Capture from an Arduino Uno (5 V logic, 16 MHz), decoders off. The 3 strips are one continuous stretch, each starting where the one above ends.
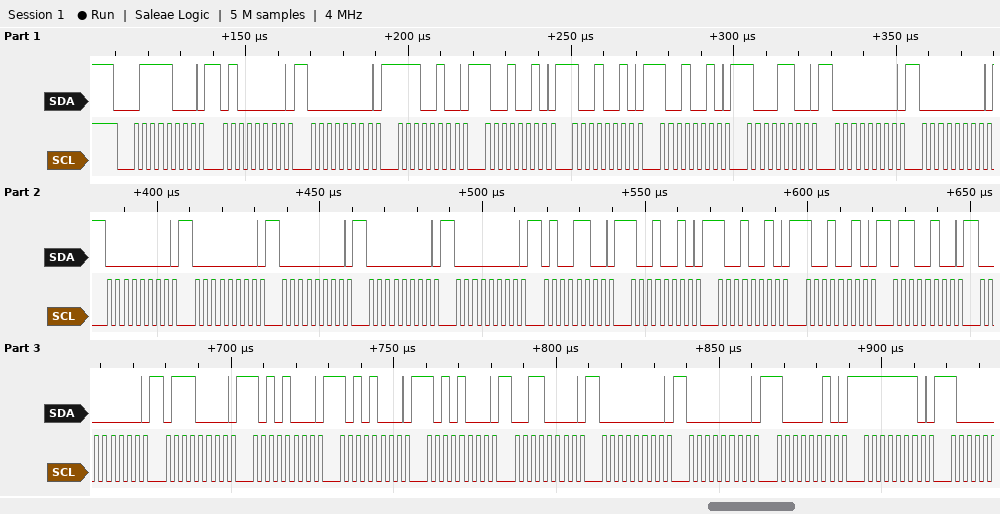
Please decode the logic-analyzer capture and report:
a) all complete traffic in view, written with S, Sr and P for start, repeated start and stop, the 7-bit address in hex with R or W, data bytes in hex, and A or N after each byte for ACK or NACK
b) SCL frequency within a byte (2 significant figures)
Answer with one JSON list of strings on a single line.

["S 3CW A 40 A 00 A E4 A 92 A 92 A 92 A 8C A 00 A 00 A 00 A 00 A 00 A 00 A 00 A 4C A 92 A 92 A 92 A 64 A 00 A 70 A A8 A A8 A A8 A 30 A 00 A 00 A 82 A FE A", "400 kHz"]
